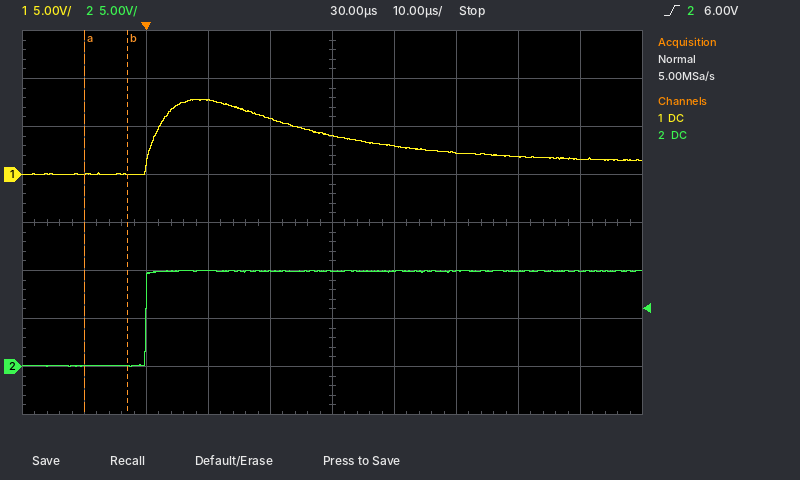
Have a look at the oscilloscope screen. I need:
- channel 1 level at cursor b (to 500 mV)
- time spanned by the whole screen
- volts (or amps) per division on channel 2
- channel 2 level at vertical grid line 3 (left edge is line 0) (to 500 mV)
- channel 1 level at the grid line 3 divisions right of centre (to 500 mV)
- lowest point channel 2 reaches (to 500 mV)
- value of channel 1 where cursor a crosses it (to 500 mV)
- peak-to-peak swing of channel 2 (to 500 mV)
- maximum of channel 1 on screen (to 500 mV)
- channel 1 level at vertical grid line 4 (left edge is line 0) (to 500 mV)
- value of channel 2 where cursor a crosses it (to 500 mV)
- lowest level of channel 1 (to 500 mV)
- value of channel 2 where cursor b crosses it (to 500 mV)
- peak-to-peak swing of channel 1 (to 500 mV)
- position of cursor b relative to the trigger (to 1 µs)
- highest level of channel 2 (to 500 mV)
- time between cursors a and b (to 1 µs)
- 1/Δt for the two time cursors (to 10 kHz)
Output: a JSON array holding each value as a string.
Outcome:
["0.0 V", "100 µs", "5 V", "10.0 V", "2.0 V", "0.0 V", "0.0 V", "10.0 V", "8.0 V", "6.0 V", "0.0 V", "0.0 V", "0.0 V", "8.0 V", "-3 µs", "10.0 V", "7 µs", "140 kHz"]
